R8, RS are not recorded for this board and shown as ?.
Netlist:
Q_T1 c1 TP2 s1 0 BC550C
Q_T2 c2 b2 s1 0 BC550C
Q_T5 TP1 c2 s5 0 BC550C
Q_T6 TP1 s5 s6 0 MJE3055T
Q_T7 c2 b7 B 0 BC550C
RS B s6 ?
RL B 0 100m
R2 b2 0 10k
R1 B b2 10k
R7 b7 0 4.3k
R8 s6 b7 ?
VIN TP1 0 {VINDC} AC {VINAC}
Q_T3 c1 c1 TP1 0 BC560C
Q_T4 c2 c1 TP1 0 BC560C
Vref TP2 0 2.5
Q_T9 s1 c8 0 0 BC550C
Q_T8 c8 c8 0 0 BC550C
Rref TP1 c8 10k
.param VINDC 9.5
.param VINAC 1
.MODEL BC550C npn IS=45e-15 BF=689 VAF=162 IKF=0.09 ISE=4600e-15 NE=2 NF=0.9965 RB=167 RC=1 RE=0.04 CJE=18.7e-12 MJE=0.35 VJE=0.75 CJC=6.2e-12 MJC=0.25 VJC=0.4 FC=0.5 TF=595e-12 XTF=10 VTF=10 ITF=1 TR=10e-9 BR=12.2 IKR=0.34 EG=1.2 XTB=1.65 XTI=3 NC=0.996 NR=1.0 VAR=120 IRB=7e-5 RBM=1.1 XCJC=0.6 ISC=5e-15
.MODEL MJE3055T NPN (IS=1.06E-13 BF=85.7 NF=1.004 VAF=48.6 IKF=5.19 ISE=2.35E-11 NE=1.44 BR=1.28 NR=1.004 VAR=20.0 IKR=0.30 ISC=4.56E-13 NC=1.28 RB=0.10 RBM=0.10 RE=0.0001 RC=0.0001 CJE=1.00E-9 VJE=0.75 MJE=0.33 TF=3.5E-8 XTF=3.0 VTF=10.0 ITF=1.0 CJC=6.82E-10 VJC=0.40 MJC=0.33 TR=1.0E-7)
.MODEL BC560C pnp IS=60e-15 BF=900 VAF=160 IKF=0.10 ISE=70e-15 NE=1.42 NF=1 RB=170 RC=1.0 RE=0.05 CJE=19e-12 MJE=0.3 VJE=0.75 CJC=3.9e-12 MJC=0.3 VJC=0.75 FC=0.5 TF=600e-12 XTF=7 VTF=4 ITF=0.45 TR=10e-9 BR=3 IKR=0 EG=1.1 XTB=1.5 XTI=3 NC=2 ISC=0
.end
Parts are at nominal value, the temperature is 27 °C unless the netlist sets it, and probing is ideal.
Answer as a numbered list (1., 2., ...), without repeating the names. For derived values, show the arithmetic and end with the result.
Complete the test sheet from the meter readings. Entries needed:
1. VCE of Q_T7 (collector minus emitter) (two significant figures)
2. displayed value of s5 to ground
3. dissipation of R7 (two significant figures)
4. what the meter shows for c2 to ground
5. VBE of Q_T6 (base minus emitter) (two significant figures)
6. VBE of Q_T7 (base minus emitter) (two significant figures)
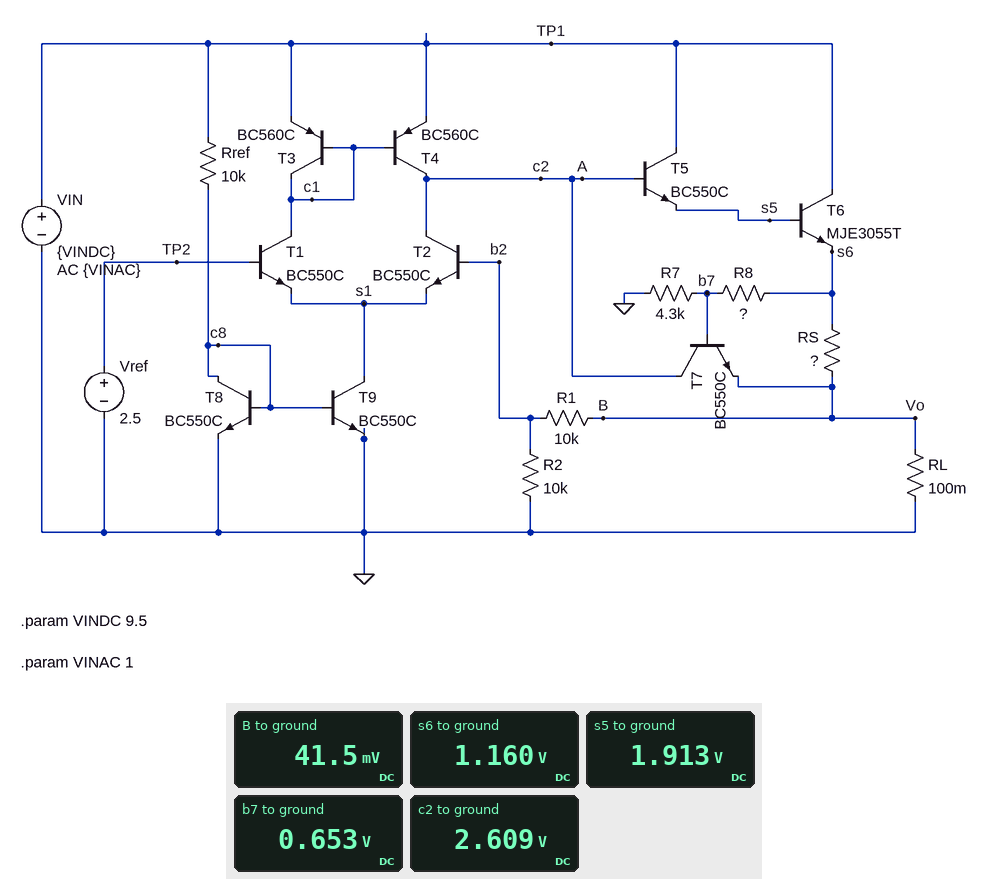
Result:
1. 2.609 V - 41.5 mV = 2.6 V
2. 1.913 V
3. (653 mV)^2 / 4.3 kΩ = 99 µW
4. 2.609 V
5. 1.913 V - 1.16 V = 750 mV
6. 653 mV - 41.5 mV = 610 mV
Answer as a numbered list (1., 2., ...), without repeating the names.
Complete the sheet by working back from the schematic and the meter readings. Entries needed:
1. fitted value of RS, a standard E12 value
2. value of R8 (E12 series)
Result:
1. 2.7 Ω
2. 3.3 kΩ
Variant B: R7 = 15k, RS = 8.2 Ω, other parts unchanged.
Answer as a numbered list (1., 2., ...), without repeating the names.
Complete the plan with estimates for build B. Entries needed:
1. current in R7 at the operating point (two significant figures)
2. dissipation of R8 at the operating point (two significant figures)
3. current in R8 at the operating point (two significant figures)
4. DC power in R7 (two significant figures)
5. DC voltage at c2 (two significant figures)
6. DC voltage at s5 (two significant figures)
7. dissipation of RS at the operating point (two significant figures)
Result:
1. 41 µA
2. 6.2 µW
3. 43 µA
4. 26 µW
5. 2.1 V
6. 1.5 V
7. 70 mW
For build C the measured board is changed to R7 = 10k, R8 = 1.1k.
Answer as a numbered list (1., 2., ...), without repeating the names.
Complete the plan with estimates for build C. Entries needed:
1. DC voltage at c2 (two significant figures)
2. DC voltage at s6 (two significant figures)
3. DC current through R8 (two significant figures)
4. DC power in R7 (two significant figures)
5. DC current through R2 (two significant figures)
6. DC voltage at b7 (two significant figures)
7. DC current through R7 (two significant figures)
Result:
1. 2.1 V
2. 710 mV
3. 66 µA
4. 41 µW
5. 1.3 µA
6. 640 mV
7. 64 µA
